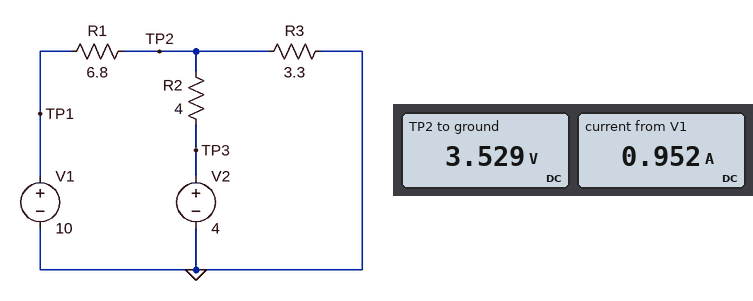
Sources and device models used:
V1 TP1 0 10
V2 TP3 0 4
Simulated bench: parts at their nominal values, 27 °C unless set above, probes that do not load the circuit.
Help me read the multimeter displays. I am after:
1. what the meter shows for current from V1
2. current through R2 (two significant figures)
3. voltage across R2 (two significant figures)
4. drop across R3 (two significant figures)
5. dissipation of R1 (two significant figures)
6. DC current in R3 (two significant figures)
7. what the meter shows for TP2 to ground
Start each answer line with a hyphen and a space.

- 0.952 A
- 120 mA
- 470 mV
- 3.5 V
- 6.2 W
- 1.1 A
- 3.529 V
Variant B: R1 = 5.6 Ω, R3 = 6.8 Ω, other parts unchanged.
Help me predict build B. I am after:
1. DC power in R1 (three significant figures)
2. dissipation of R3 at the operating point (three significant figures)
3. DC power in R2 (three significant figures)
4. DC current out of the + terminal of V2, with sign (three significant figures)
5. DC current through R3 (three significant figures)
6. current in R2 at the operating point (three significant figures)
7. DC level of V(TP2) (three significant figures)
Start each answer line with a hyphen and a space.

- 4.76 W
- 3.44 W
- 176 mW
- -210 mA
- 712 mA
- 210 mA
- 4.84 V
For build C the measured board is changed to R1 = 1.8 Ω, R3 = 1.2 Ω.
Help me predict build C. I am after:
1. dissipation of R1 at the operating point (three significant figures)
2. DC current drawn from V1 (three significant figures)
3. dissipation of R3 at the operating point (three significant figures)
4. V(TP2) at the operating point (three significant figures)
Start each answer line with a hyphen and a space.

- 20.0 W
- 3.33 A
- 13.3 W
- 4.00 V
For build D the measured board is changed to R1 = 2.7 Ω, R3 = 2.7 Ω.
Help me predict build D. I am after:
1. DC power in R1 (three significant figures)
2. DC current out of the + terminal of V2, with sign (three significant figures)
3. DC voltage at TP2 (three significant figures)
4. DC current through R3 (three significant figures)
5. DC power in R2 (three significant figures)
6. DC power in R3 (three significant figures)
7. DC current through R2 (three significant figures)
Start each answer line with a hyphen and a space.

- 10.2 W
- -187 mA
- 4.75 V
- 1.76 A
- 140 mW
- 8.35 W
- 187 mA
